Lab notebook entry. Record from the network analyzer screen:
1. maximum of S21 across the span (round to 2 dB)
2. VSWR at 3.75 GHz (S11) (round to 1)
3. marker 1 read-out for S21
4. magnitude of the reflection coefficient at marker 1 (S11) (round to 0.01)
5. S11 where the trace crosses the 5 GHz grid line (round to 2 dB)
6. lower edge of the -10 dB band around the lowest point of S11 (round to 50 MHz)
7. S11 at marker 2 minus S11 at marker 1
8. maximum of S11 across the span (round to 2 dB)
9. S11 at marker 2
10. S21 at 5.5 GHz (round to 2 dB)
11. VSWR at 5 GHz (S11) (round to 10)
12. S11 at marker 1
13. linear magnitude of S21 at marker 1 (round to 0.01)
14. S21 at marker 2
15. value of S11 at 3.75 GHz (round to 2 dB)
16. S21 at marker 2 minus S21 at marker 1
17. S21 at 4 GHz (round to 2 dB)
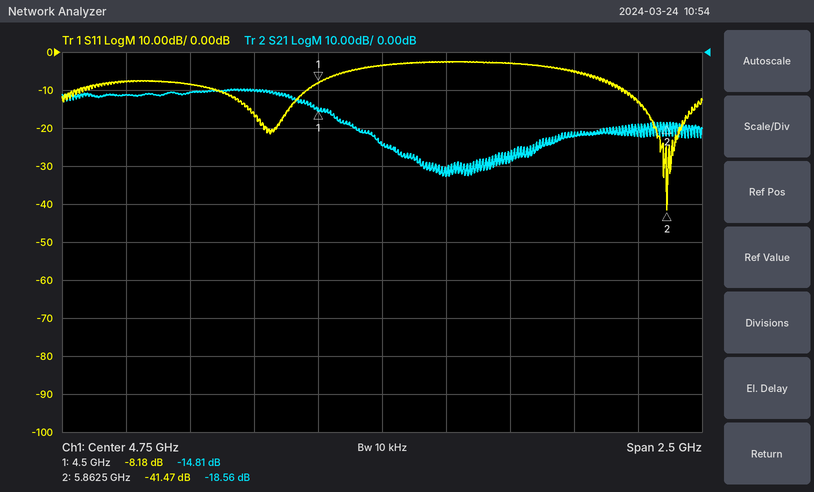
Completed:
-10 dB
2
-14.81 dB
0.39
-2 dB
5.70 GHz
-33.29 dB
-2 dB
-41.47 dB
-22 dB
10
-8.18 dB
0.18
-18.56 dB
-8 dB
-3.75 dB
-10 dB
